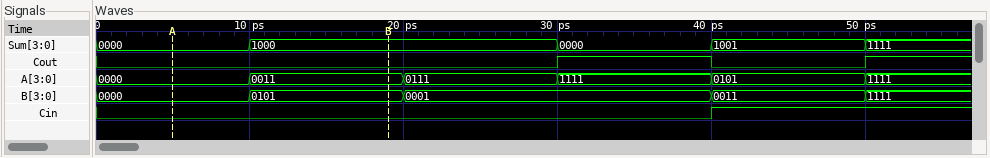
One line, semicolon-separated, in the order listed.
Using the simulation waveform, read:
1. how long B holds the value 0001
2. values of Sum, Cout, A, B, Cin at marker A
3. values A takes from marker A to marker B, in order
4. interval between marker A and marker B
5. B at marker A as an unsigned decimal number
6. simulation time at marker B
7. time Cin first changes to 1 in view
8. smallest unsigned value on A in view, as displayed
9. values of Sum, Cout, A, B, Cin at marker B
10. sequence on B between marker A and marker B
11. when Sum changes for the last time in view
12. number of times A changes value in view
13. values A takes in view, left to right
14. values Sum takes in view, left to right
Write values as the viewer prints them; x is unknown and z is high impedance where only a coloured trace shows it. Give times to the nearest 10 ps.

20 ps; Sum=0000, Cout=0, A=0000, B=0000, Cin=0; 0000, 0011; 10 ps; 0; 20 ps; 40 ps; 0000; Sum=1000, Cout=0, A=0011, B=0101, Cin=0; 0000, 0101; 50 ps; 5; 0000, 0011, 0111, 1111, 0101, 1111; 0000, 1000, 0000, 1001, 1111
